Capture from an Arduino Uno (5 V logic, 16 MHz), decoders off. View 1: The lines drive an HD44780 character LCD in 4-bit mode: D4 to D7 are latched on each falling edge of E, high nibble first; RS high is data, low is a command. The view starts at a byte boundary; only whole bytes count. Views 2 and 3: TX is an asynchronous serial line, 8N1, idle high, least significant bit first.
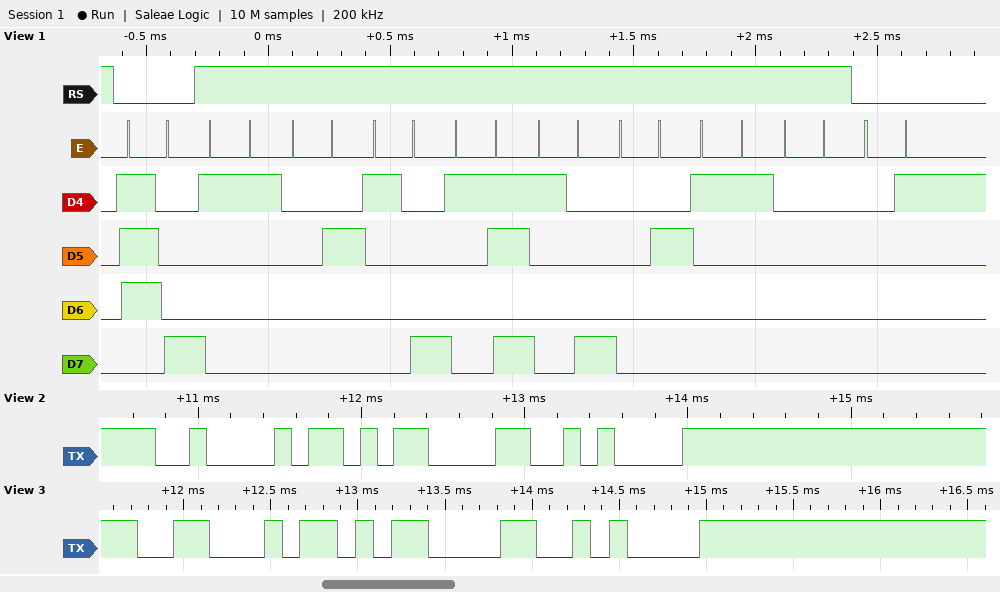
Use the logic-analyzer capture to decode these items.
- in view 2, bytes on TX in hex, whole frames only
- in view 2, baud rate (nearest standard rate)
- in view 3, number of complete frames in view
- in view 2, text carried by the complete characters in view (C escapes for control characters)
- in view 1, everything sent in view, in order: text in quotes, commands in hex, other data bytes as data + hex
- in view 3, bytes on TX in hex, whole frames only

42 0D 0A
9600 baud
3
"B\r\n"
0x78 data 11 02 18 1B 18 02 11 00 0x01
46 0D 0A
